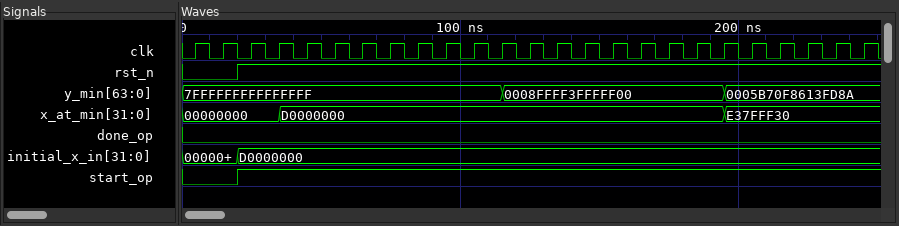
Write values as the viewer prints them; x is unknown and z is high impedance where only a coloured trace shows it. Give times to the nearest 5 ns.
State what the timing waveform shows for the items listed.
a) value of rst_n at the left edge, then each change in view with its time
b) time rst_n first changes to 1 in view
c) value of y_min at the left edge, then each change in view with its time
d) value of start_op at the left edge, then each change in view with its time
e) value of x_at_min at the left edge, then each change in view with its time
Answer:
0, 1 at 20 ns
20 ns
7FFFFFFFFFFFFFFF, 0008FFFF3FFFFF00 at 115 ns, 0005B70F8613FD8A at 195 ns
0, 1 at 20 ns
00000000, D0000000 at 35 ns, E37FFF30 at 195 ns
